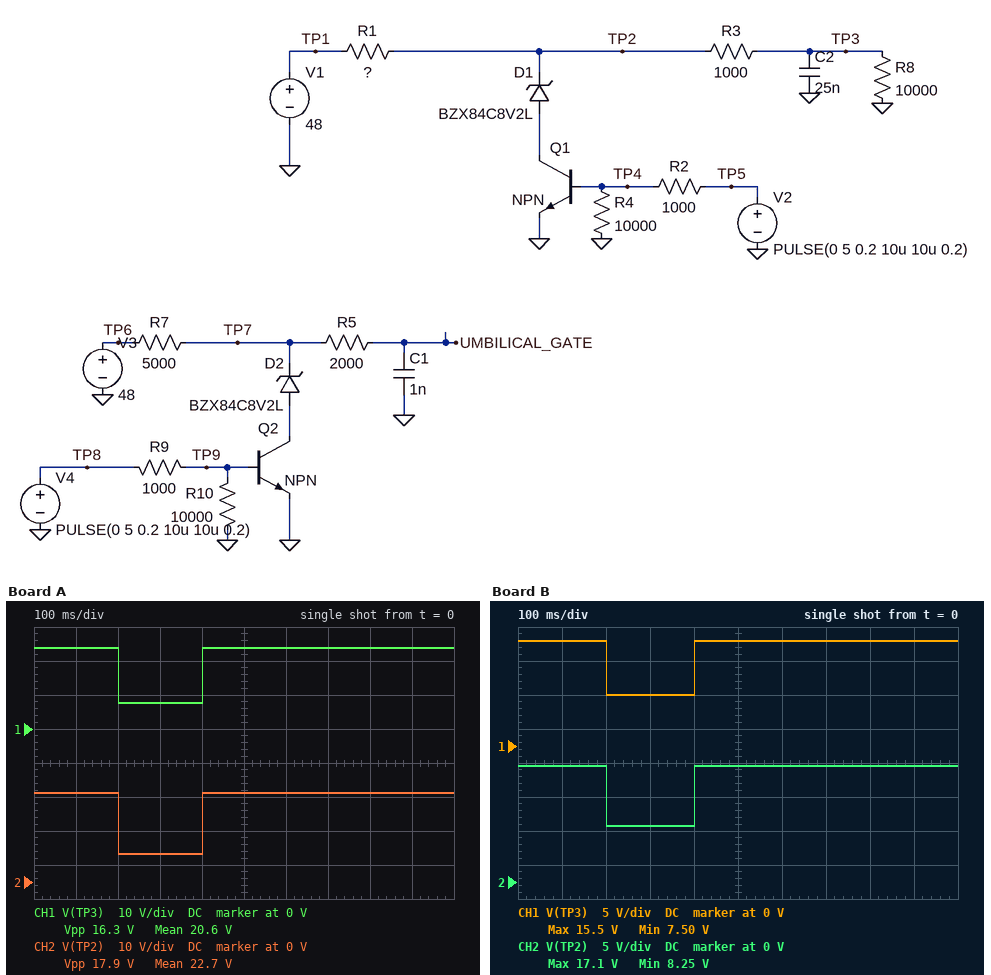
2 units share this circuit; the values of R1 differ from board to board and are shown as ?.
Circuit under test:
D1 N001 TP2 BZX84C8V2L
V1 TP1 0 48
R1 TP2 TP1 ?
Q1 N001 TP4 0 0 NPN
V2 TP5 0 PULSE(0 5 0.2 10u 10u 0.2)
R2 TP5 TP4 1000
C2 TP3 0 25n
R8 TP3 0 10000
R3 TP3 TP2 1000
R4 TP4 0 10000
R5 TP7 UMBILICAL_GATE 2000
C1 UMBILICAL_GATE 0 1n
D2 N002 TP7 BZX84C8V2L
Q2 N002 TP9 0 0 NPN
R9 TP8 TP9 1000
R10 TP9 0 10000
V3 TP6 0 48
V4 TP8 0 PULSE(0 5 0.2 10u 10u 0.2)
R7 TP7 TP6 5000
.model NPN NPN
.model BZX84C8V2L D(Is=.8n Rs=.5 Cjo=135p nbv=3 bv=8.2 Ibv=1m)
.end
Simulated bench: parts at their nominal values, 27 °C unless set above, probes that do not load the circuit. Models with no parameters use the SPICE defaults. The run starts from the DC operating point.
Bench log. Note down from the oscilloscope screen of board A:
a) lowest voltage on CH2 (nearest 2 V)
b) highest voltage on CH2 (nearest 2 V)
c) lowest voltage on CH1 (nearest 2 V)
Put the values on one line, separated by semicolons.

8 V; 26 V; 8 V
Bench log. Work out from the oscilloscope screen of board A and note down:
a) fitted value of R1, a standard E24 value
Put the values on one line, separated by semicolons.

9.1 kΩ
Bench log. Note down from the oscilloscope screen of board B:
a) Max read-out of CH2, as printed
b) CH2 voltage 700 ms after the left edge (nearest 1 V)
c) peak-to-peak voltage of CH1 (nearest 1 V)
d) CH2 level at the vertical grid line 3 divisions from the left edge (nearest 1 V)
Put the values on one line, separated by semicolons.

17.1 V; 17 V; 8 V; 8 V
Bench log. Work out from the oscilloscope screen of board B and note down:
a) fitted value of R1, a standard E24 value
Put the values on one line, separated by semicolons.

20 kΩ
